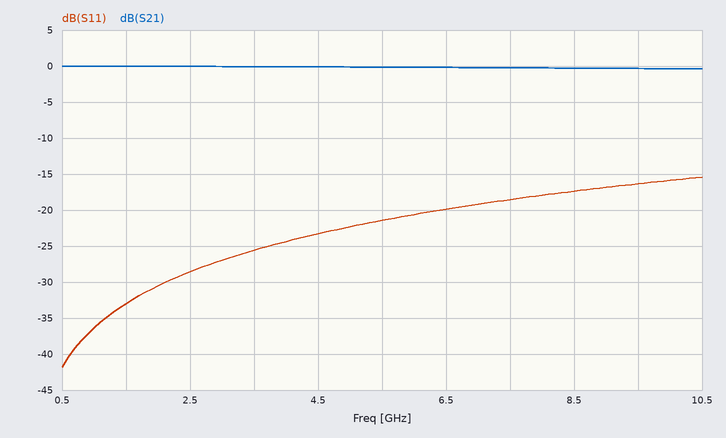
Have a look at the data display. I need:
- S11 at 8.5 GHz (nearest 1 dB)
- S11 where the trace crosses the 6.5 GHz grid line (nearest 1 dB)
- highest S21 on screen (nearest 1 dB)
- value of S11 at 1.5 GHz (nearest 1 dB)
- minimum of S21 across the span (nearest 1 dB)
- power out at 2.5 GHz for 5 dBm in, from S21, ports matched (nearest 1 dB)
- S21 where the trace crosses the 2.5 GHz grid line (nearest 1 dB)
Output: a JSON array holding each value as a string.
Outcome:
["-17 dB", "-20 dB", "0 dB", "-33 dB", "0 dB", "5 dBm", "0 dB"]
